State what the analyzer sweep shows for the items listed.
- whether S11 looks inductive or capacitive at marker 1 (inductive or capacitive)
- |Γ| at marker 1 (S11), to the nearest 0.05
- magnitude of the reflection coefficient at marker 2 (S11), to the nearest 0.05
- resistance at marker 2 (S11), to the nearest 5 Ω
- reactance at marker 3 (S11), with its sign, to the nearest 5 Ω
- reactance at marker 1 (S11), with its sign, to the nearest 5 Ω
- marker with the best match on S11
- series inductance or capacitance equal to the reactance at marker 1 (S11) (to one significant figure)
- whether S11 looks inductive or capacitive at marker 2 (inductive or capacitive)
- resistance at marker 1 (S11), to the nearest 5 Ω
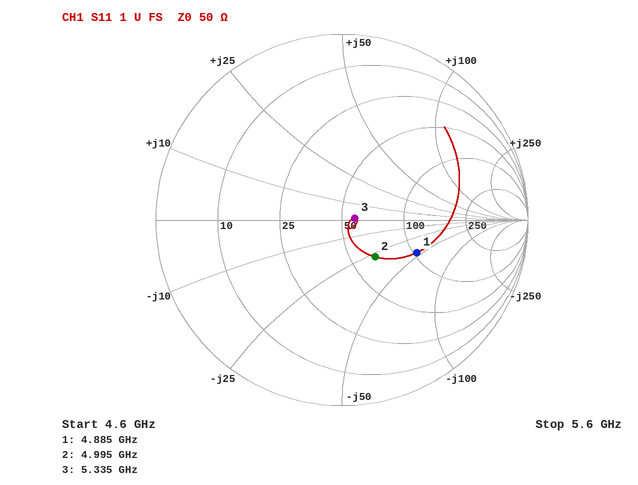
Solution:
capacitive
0.45
0.25
65 Ω
0 Ω
-45 Ω
marker 3
700 fF
capacitive
105 Ω
